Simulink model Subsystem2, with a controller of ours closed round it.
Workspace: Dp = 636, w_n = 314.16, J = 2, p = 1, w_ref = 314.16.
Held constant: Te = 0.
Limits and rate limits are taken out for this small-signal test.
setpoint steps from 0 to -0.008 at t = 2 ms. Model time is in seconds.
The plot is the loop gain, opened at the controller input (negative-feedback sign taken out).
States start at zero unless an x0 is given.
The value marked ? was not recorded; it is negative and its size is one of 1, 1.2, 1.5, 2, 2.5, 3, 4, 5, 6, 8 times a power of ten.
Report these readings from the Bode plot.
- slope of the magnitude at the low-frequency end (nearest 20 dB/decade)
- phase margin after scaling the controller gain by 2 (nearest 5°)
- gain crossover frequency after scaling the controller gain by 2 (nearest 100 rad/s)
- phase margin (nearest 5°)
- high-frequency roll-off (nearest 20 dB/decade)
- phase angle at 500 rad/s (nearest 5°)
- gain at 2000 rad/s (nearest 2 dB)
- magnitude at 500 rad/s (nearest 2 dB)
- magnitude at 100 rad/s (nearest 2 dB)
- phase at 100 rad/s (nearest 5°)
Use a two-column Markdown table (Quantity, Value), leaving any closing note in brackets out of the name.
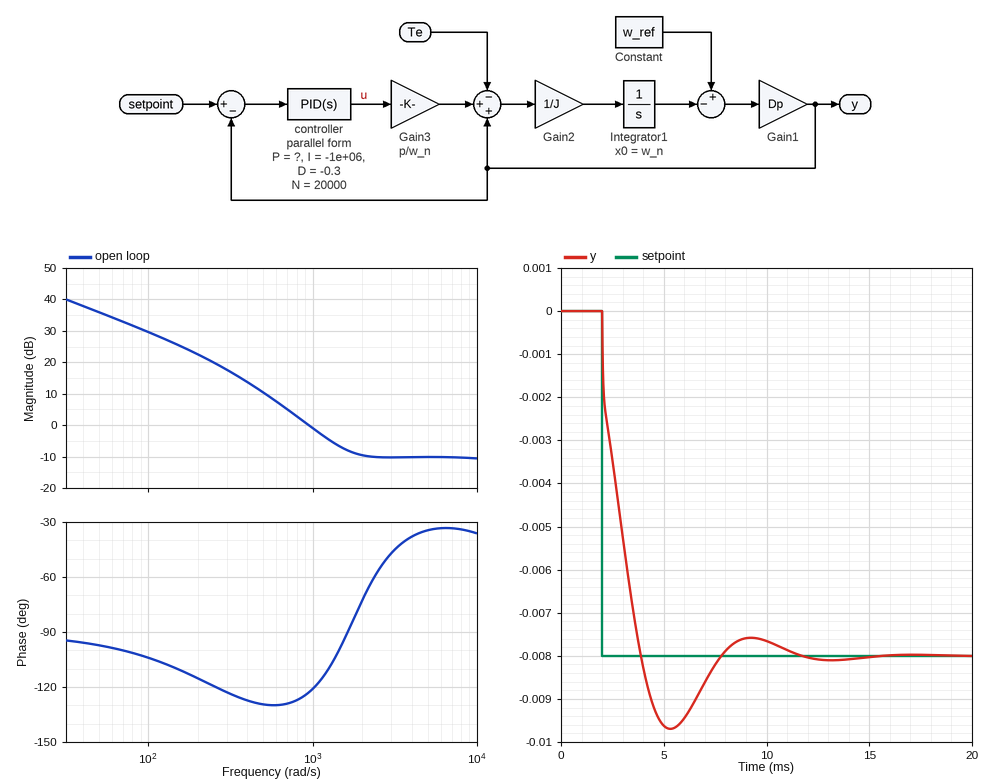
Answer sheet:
| Quantity | Value |
|---|---|
| slope of the magnitude at the low-frequency end | -20 dB/decade |
| phase margin after scaling the controller gain by 2 | 75° |
| gain crossover frequency after scaling the controller gain by 2 | 1400 rad/s |
| phase margin | 55° |
| high-frequency roll-off | 0 dB/decade |
| phase angle at 500 rad/s | -130° |
| gain at 2000 rad/s | -10 dB |
| magnitude at 500 rad/s | 10 dB |
| magnitude at 100 rad/s | 30 dB |
| phase at 100 rad/s | -105° |
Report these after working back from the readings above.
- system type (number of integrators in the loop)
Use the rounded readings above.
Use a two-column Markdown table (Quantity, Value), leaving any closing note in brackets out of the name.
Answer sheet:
| Quantity | Value |
|---|---|
| system type | 1 |
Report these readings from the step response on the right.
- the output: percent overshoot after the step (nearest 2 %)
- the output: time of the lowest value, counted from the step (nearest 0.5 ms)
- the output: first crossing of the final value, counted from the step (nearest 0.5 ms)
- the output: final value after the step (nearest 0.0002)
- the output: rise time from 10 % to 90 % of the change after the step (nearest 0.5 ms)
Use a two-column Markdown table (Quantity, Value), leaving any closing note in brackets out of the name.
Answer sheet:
| Quantity | Value |
|---|---|
| the output: percent overshoot after the step | 22 % |
| the output: time of the lowest value, counted from the step | 3.5 ms |
| the output: first crossing of the final value, counted from the step | 2.0 ms |
| the output: final value after the step | -0.0080 |
| the output: rise time from 10 % to 90 % of the change after the step | 1.5 ms |
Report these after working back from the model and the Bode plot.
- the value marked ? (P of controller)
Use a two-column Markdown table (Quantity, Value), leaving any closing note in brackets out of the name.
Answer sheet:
| Quantity | Value |
|---|---|
| the value marked ? | -600 |
